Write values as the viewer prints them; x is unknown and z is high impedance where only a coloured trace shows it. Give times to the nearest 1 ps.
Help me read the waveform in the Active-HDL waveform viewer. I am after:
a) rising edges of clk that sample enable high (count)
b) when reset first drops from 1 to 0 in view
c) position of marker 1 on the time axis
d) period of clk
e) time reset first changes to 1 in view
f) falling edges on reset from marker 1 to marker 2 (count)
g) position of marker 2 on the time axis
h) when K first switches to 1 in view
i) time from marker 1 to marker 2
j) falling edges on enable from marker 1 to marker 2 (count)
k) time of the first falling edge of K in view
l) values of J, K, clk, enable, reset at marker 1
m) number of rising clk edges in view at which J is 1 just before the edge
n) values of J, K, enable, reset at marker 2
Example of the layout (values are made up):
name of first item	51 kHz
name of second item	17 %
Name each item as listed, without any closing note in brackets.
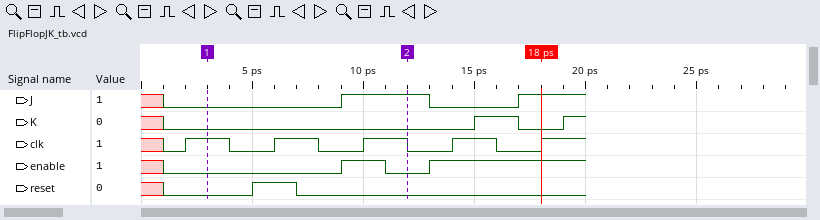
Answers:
rising edges of clk that sample enable high	3
when reset first drops from 1 to 0 in view	7 ps
position of marker 1 on the time axis	3 ps
period of clk	4 ps
time reset first changes to 1 in view	5 ps
falling edges on reset from marker 1 to marker 2	1
position of marker 2 on the time axis	12 ps
when K first switches to 1 in view	15 ps
time from marker 1 to marker 2	9 ps
falling edges on enable from marker 1 to marker 2	1
time of the first falling edge of K in view	17 ps
values of J, K, clk, enable, reset at marker 1	J=0, K=0, clk=1, enable=0, reset=0
number of rising clk edges in view at which J is 1 just before the edge	2
values of J, K, enable, reset at marker 2	J=1, K=0, enable=0, reset=0
